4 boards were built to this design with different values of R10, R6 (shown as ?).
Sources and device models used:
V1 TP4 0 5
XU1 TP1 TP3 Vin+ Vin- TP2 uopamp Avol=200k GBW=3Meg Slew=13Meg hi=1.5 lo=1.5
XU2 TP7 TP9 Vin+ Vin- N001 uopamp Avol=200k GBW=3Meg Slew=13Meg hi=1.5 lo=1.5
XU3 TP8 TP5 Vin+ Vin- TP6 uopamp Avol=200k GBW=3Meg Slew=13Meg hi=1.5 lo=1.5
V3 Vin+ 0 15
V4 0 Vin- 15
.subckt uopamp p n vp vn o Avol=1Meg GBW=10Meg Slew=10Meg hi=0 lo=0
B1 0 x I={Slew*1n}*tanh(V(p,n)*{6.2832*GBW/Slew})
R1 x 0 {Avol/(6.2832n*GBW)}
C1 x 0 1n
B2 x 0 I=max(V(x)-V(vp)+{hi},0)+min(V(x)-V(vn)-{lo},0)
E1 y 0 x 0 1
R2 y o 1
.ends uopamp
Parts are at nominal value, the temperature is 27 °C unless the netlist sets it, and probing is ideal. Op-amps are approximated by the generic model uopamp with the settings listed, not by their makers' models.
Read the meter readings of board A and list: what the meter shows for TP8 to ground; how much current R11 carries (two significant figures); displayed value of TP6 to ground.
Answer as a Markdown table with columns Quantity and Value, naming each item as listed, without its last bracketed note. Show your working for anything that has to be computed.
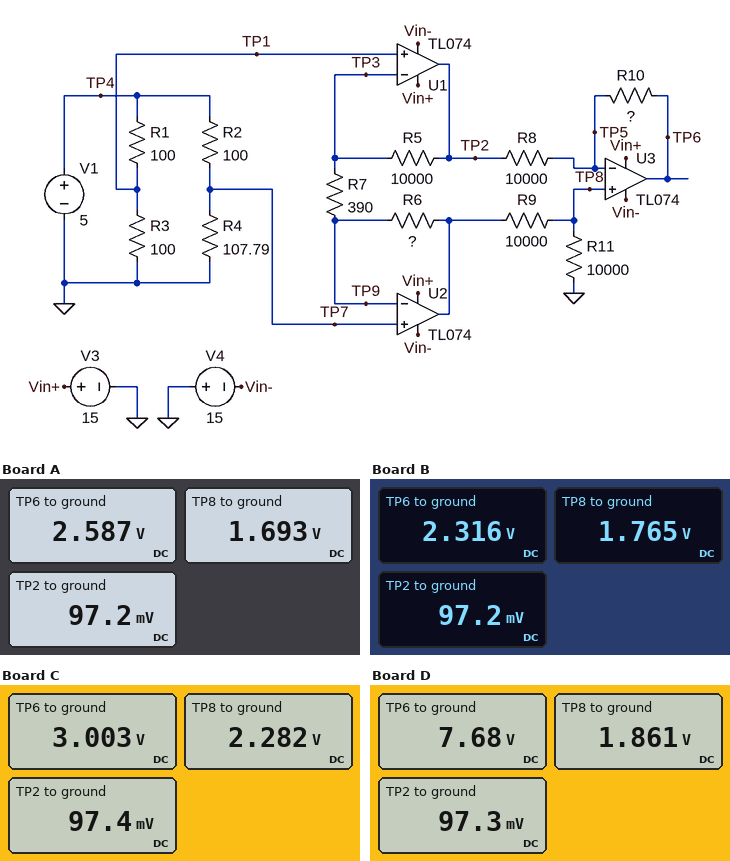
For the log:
| Quantity | Value |
|---|---|
| what the meter shows for TP8 to ground | 1.693 V |
| how much current R11 carries | (1.693 V) / 10 kΩ = 170 µA |
| displayed value of TP6 to ground | 2.587 V |
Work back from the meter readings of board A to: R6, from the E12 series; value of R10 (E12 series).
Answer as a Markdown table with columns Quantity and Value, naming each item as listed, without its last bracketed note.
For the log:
| Quantity | Value |
|---|---|
| R6, from the E12 series | 3.3 kΩ |
| value of R10 | 5.6 kΩ |
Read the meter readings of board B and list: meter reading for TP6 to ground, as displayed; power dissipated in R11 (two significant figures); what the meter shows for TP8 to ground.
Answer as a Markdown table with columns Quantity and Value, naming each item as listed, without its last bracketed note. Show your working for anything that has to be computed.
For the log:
| Quantity | Value |
|---|---|
| meter reading for TP6 to ground, as displayed | 2.316 V |
| power dissipated in R11 | (1.765 V)^2 / 10 kΩ = 310 µW |
| what the meter shows for TP8 to ground | 1.765 V |
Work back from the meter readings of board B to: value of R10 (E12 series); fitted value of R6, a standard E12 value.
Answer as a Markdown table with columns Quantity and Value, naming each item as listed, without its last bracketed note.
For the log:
| Quantity | Value |
|---|---|
| value of R10 | 3.3 kΩ |
| fitted value of R6, a standard E12 value | 3.9 kΩ |
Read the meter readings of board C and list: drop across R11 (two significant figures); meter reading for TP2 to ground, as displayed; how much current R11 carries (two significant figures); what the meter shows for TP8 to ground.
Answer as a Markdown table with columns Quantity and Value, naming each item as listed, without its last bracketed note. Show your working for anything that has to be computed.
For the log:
| Quantity | Value |
|---|---|
| drop across R11 | 2.282 V = 2.3 V |
| meter reading for TP2 to ground, as displayed | 97.4 mV |
| how much current R11 carries | (2.282 V) / 10 kΩ = 230 µA |
| what the meter shows for TP8 to ground | 2.282 V |
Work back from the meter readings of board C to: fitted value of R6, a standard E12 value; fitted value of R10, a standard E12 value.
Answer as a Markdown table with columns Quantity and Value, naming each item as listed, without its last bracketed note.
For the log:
| Quantity | Value |
|---|---|
| fitted value of R6, a standard E12 value | 8.2 kΩ |
| fitted value of R10, a standard E12 value | 3.3 kΩ |
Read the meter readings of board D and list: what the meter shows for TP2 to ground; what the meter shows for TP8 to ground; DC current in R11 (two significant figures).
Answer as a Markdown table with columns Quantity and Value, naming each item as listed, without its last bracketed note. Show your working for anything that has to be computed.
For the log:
| Quantity | Value |
|---|---|
| what the meter shows for TP2 to ground | 97.3 mV |
| what the meter shows for TP8 to ground | 1.861 V |
| DC current in R11 | (1.861 V) / 10 kΩ = 190 µA |
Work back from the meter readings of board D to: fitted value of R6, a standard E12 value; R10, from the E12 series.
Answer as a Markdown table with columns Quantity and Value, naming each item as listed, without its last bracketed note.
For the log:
| Quantity | Value |
|---|---|
| fitted value of R6, a standard E12 value | 4.7 kΩ |
| R10, from the E12 series | 33 kΩ |
